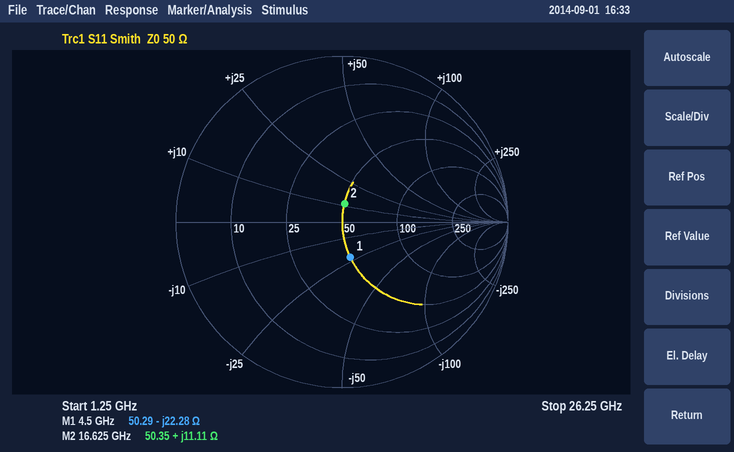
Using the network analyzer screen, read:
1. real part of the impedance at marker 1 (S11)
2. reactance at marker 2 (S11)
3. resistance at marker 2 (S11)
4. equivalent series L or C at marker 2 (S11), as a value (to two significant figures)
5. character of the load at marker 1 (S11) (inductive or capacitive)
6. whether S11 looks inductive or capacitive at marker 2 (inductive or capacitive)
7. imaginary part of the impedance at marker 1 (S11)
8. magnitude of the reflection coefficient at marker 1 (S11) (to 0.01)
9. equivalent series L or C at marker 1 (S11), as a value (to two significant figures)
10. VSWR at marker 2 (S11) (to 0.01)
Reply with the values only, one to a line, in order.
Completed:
50.29 Ω
+11.11 Ω
50.35 Ω
110 pH
capacitive
inductive
-22.28 Ω
0.22
1.6 pF
1.25
